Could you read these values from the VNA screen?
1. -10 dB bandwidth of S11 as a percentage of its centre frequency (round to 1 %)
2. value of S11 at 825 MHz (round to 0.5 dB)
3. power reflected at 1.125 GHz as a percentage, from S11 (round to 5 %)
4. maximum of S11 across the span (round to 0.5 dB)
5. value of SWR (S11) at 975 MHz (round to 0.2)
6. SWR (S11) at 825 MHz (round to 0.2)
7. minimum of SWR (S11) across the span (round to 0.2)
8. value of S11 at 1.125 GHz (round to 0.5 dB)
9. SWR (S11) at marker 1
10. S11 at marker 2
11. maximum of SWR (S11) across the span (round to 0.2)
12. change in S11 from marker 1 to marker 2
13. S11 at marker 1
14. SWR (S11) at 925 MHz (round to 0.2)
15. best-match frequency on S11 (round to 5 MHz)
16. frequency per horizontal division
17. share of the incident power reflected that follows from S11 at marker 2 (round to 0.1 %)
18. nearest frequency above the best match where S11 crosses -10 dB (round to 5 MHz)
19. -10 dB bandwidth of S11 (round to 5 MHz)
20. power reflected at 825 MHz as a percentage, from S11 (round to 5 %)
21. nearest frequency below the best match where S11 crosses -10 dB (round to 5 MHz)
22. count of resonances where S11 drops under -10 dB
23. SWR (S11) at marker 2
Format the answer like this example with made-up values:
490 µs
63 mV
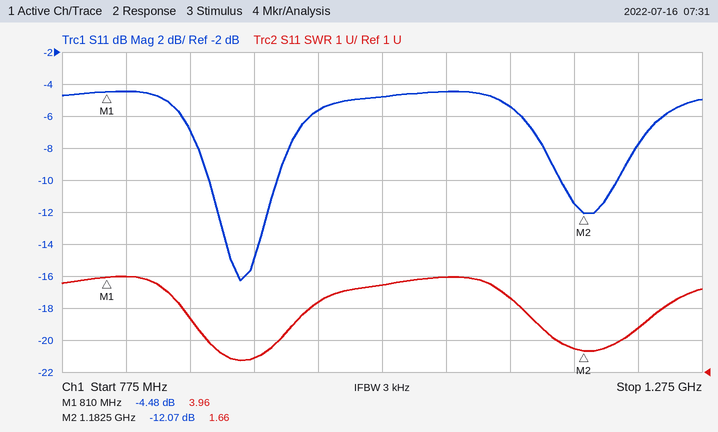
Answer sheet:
6 %
-4.5 dB
30 %
-4.5 dB
3.2
4.0
1.4
-5.5 dB
3.96
-12.07 dB
4.0
-7.59 dB
-4.48 dB
1.4
915 MHz
50 MHz
6.2 %
945 MHz
55 MHz
35 %
890 MHz
2
1.66
